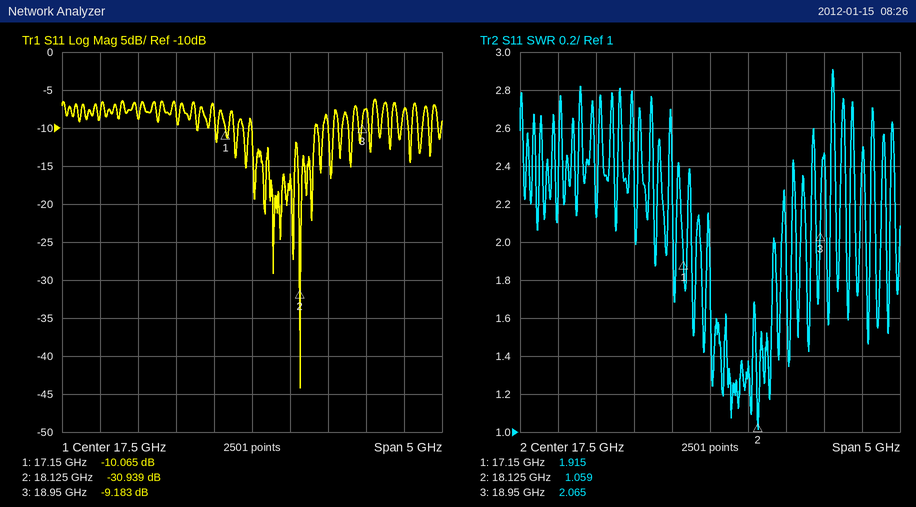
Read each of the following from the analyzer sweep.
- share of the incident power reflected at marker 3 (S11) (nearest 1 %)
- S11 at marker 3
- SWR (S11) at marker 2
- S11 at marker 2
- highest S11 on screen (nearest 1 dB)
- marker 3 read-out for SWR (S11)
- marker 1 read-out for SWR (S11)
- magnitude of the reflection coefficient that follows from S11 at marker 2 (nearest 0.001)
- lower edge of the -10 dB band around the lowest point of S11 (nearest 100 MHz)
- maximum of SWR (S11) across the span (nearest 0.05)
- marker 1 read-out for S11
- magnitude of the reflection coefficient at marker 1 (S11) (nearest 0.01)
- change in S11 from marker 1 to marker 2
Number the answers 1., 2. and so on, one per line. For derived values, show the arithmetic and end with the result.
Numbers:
1. 10^(-9.183/10) ≈ 12 %
2. -9.183 dB
3. 1.059
4. -30.939 dB
5. -6 dB
6. 2.065
7. 1.915
8. 10^(-30.939/20) ≈ 0.028
9. 17.5 GHz
10. 2.90
11. -10.065 dB
12. 10^(-10.065/20) ≈ 0.31
13. -30.939 − (-10.065) = -20.874 dB
